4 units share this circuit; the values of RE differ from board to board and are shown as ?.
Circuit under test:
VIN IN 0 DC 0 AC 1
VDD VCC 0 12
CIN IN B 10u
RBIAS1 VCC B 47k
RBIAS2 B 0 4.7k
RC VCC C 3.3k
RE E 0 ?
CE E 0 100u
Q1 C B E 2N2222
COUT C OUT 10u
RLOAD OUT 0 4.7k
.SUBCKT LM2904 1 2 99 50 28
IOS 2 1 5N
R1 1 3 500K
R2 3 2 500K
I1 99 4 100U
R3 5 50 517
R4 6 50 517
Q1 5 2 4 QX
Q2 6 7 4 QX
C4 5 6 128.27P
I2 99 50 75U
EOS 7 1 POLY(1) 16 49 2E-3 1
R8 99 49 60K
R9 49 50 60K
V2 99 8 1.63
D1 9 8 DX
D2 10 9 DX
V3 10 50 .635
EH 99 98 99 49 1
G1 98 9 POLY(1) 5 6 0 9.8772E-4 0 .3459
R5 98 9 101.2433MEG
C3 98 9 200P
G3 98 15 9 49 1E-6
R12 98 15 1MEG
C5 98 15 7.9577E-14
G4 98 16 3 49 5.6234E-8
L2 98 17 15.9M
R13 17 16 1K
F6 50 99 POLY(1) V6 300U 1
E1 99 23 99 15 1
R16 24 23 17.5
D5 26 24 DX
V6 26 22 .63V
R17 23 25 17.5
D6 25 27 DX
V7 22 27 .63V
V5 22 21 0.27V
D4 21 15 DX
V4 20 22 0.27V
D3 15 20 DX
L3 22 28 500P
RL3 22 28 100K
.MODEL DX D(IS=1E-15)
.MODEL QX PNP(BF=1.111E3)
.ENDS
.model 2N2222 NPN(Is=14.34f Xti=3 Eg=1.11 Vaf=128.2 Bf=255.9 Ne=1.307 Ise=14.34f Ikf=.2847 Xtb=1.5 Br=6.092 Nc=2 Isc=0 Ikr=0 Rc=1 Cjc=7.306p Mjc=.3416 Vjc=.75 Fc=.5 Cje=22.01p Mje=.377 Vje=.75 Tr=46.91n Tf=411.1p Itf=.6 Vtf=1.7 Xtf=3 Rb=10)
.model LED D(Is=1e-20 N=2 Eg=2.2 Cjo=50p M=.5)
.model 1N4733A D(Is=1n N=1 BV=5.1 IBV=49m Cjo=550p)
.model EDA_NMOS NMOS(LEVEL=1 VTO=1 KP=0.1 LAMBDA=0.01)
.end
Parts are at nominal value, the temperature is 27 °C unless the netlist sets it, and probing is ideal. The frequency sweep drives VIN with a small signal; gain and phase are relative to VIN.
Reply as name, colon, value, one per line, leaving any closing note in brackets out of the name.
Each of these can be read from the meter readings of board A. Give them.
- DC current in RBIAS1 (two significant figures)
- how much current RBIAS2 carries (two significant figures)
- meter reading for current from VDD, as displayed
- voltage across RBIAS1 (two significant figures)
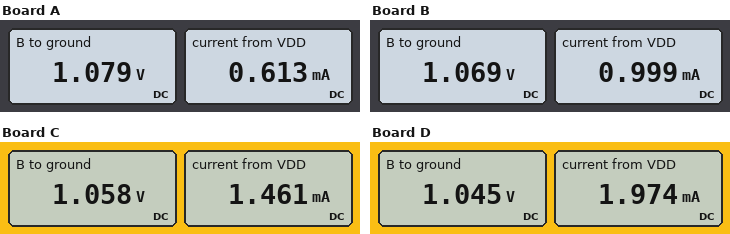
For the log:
DC current in RBIAS1: 230 µA
how much current RBIAS2 carries: 230 µA
meter reading for current from VDD, as displayed: 0.613 mA
voltage across RBIAS1: 11 V
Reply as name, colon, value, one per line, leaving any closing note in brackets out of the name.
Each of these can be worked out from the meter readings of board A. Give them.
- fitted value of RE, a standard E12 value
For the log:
fitted value of RE, a standard E12 value: 1.2 kΩ
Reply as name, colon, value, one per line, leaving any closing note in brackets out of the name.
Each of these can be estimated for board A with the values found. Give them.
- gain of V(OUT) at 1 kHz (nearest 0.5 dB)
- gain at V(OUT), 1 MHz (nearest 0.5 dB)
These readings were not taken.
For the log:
gain of V(OUT) at 1 kHz: 29.0 dB
gain at V(OUT), 1 MHz: 29.0 dB
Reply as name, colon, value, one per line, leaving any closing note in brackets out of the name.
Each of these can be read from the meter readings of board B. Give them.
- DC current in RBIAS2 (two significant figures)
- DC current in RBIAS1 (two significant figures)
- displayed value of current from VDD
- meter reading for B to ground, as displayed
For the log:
DC current in RBIAS2: 230 µA
DC current in RBIAS1: 230 µA
displayed value of current from VDD: 0.999 mA
meter reading for B to ground, as displayed: 1.069 V
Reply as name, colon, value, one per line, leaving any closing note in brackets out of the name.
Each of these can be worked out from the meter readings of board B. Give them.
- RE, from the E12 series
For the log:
RE, from the E12 series: 560 Ω
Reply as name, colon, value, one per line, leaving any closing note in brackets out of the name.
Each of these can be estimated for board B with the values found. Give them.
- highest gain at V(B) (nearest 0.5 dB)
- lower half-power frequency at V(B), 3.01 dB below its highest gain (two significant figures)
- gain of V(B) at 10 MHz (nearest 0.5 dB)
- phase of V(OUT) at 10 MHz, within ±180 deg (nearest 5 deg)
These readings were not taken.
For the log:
highest gain at V(B): 0 dB
lower half-power frequency at V(B), 3.01 dB below its highest gain: 4.1 Hz
gain of V(B) at 10 MHz: 0 dB
phase of V(OUT) at 10 MHz, within ±180 deg: 150 deg
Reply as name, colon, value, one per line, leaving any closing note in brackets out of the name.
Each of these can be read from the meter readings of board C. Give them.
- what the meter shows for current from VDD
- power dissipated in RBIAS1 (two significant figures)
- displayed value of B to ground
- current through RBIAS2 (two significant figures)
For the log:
what the meter shows for current from VDD: 1.461 mA
power dissipated in RBIAS1: 2.5 mW
displayed value of B to ground: 1.058 V
current through RBIAS2: 230 µA
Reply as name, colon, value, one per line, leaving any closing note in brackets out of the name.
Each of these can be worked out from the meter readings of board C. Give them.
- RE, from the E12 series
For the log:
RE, from the E12 series: 330 Ω
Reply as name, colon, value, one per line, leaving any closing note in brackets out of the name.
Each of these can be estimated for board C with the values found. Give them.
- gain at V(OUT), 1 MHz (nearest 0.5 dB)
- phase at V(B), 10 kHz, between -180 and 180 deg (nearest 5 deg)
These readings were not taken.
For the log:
gain at V(OUT), 1 MHz: 39.0 dB
phase at V(B), 10 kHz, between -180 and 180 deg: 0 deg
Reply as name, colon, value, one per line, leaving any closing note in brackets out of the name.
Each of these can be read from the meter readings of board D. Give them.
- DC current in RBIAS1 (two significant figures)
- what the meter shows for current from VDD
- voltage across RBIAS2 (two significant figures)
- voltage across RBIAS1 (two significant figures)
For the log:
DC current in RBIAS1: 230 µA
what the meter shows for current from VDD: 1.974 mA
voltage across RBIAS2: 1.0 V
voltage across RBIAS1: 11 V
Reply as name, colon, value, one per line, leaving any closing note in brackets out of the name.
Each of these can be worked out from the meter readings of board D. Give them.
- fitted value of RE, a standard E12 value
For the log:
fitted value of RE, a standard E12 value: 220 Ω
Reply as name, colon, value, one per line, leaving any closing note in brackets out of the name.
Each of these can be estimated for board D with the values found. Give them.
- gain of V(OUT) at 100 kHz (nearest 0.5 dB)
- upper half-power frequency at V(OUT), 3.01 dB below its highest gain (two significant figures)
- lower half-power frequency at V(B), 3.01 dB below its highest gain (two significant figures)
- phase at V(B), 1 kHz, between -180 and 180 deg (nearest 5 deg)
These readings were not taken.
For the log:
gain of V(OUT) at 100 kHz: 42.0 dB
upper half-power frequency at V(OUT), 3.01 dB below its highest gain: 14 MHz
lower half-power frequency at V(B), 3.01 dB below its highest gain: 4.4 Hz
phase at V(B), 1 kHz, between -180 and 180 deg: 0 deg
